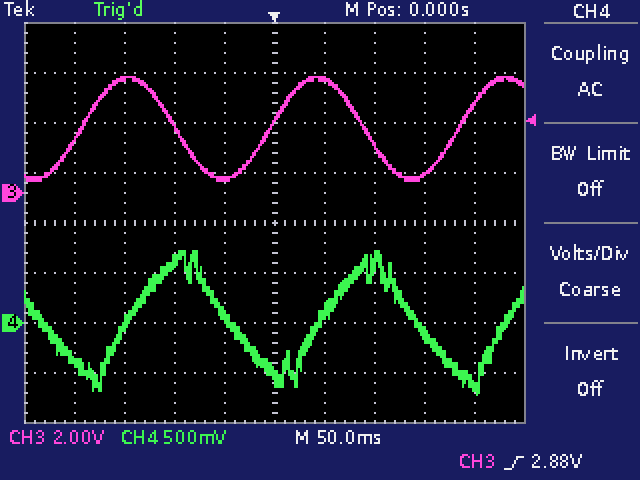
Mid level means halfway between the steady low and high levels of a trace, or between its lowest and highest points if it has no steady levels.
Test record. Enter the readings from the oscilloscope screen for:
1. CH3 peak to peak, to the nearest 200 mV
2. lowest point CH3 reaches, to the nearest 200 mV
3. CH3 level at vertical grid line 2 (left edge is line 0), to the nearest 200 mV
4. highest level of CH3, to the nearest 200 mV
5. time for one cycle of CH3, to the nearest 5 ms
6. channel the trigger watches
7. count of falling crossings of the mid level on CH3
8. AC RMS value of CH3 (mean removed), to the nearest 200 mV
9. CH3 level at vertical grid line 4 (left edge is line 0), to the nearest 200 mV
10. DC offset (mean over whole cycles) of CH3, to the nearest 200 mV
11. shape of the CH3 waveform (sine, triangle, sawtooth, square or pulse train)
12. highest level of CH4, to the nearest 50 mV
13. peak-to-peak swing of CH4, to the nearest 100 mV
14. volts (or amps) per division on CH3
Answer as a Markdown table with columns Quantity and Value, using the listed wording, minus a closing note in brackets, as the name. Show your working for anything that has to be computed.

| Quantity | Value |
|---|---|
| CH3 peak to peak, to the nearest 200 mV | 4.6 V − (400 mV) = 4.2 V |
| lowest point CH3 reaches, to the nearest 200 mV | 400 mV |
| CH3 level at vertical grid line 2 (left edge is line 0), to the nearest 200 mV | 4.6 V |
| highest level of CH3, to the nearest 200 mV | 4.6 V |
| time for one cycle of CH3, to the nearest 5 ms | 190 ms |
| channel the trigger watches | CH3 |
| count of falling crossings of the mid level on CH3 | 2 |
| AC RMS value of CH3 (mean removed), to the nearest 200 mV | 4.2 V / (2√2) ≈ 1.48 V, so 1.4 V to the nearest 200 mV |
| CH3 level at vertical grid line 4 (left edge is line 0), to the nearest 200 mV | 600 mV |
| DC offset (mean over whole cycles) of CH3, to the nearest 200 mV | (4.6 V + (400 mV)) / 2 ≈ 2.50 V, so 2.6 V to the nearest 200 mV |
| shape of the CH3 waveform | sine |
| highest level of CH4, to the nearest 50 mV | 700 mV |
| peak-to-peak swing of CH4, to the nearest 100 mV | 1.40 V |
| volts (or amps) per division on CH3 | 2 V |
